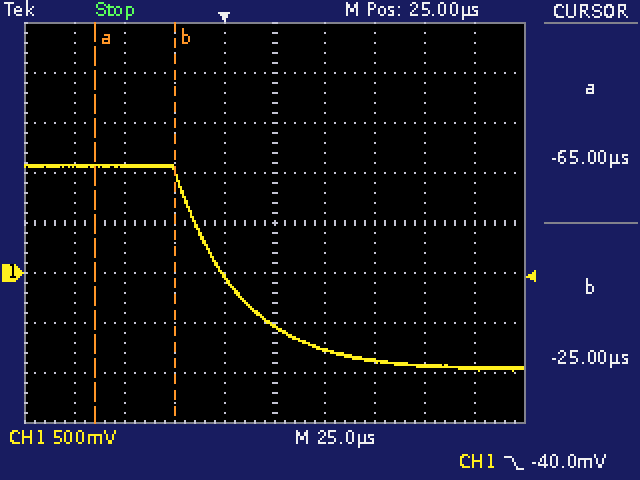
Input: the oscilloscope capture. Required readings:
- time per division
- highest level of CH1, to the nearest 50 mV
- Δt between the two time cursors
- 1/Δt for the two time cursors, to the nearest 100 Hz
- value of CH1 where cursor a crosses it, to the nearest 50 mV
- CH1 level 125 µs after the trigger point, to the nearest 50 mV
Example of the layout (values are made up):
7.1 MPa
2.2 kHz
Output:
25 µs
1.10 V
40.0 µs
25.0 kHz
1.05 V
-950 mV
